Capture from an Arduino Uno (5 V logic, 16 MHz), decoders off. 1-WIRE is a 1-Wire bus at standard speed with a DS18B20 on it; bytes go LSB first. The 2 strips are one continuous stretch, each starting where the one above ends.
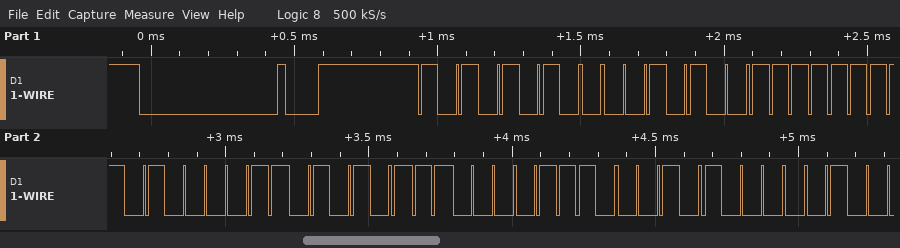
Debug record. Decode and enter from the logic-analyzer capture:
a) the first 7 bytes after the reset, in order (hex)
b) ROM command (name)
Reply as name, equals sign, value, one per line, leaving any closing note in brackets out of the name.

the first 7 bytes after the reset, in order = 55 28 FF C2 EA 70 14
ROM command = Match ROM
